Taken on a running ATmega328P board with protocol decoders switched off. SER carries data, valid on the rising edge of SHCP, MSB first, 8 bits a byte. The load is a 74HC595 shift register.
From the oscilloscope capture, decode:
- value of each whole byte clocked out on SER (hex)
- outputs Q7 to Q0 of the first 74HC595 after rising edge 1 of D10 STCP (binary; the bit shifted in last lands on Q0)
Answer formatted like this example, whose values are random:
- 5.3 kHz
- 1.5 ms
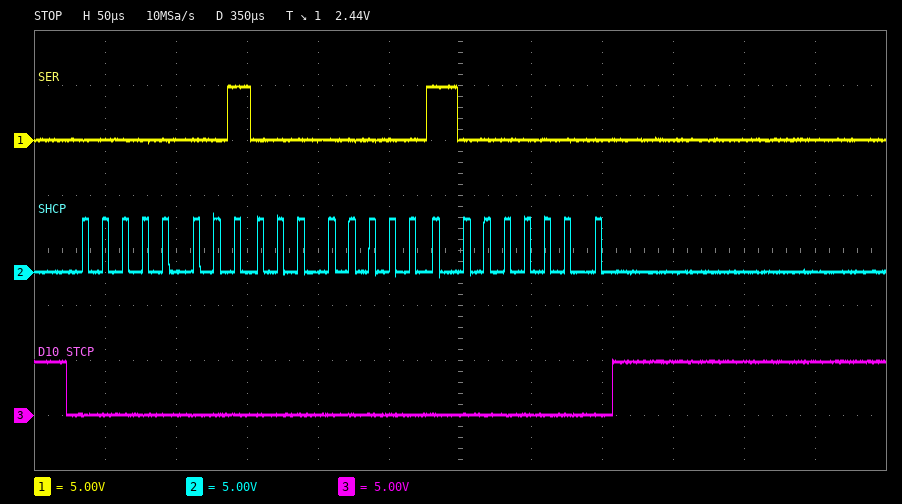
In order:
- 0x01 0x00 0x80
- 10000000
